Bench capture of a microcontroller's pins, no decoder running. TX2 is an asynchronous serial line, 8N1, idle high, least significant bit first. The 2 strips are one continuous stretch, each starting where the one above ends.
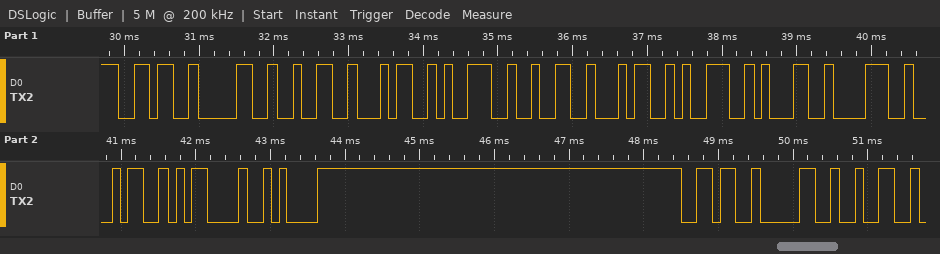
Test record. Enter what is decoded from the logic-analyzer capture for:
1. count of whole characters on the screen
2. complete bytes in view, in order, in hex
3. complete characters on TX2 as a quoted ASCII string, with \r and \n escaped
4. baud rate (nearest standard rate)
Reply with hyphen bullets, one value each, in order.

- 16
- 36 30 32 34 39 32 34 39 31 38 34 0D 0A 36 30 32
- "60249249184\r\n602"
- 9600 baud
